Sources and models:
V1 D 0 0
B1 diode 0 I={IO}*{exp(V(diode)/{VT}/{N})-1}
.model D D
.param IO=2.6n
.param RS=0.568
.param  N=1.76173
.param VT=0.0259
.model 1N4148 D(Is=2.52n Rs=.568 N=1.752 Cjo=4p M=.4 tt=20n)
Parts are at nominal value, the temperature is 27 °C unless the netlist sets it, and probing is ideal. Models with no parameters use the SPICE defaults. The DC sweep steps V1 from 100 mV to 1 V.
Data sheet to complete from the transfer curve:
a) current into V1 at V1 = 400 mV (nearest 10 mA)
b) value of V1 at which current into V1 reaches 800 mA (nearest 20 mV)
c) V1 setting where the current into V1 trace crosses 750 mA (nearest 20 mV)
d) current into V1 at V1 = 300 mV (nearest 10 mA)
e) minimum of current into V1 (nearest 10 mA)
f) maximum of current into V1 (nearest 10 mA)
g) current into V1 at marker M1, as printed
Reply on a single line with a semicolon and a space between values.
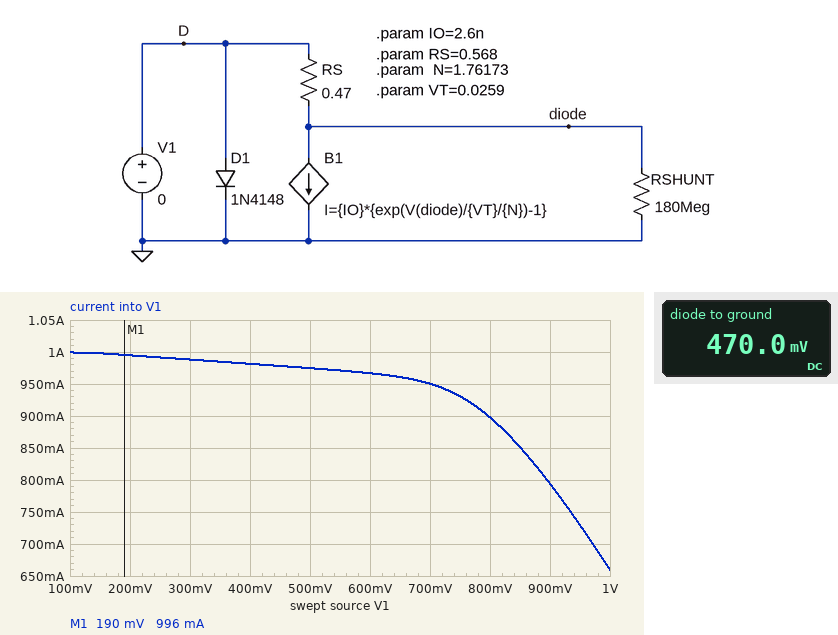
980 mA; 900 mV; 940 mV; 990 mA; 660 mA; 1.00 A; 996 mA
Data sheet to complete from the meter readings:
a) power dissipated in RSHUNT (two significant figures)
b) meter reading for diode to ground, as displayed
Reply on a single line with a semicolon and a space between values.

1.2 nW; 470.0 mV
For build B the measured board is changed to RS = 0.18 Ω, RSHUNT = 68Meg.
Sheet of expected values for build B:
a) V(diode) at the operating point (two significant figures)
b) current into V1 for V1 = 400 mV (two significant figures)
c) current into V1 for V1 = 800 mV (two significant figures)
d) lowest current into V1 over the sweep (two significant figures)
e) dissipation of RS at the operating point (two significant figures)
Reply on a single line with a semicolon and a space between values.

180 mV; 1.0 A; 920 mA; 680 mA; 180 mW
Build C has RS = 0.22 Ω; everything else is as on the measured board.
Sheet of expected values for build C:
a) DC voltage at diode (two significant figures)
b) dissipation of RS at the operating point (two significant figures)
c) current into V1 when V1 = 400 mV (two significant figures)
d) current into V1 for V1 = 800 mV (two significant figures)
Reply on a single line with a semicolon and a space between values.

220 mV; 220 mW; 1.0 A; 910 mA
